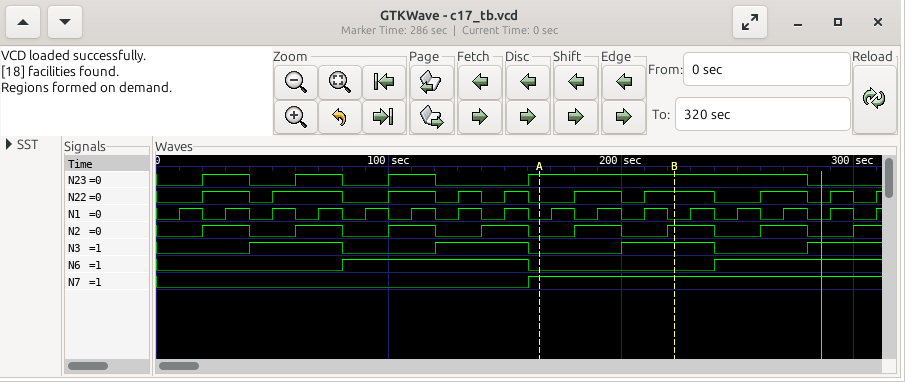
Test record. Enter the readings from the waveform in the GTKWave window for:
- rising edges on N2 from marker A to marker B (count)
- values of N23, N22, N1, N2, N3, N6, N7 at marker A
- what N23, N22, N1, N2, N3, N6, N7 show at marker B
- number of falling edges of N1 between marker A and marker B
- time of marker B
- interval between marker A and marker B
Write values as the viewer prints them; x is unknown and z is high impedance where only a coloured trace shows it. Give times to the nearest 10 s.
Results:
2
N23=1, N22=0, N1=0, N2=0, N3=0, N6=0, N7=1
N23=1, N22=1, N1=0, N2=1, N3=1, N6=0, N7=1
3
220 s
60 s
